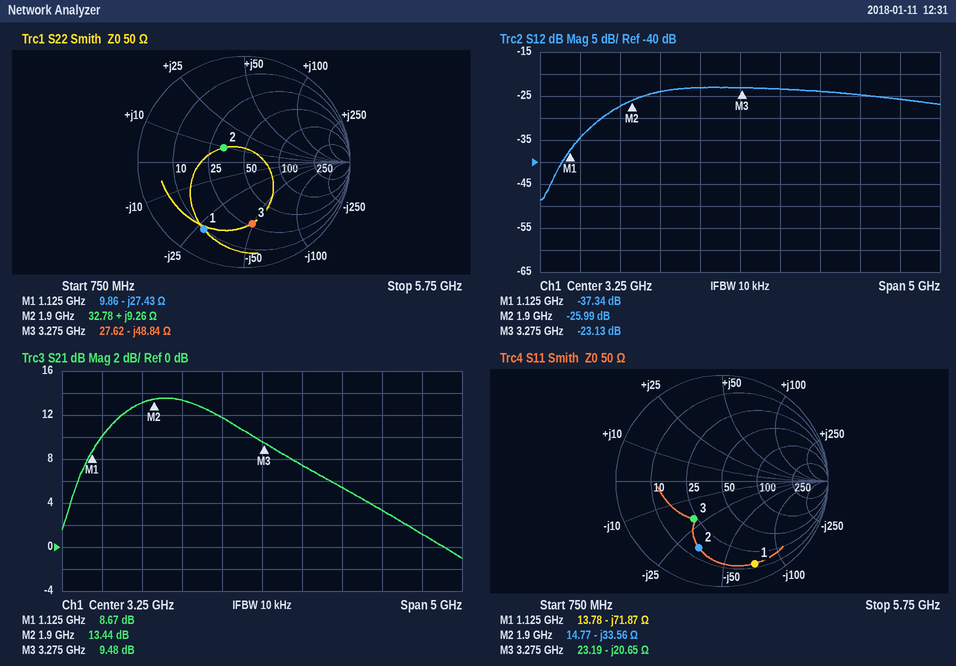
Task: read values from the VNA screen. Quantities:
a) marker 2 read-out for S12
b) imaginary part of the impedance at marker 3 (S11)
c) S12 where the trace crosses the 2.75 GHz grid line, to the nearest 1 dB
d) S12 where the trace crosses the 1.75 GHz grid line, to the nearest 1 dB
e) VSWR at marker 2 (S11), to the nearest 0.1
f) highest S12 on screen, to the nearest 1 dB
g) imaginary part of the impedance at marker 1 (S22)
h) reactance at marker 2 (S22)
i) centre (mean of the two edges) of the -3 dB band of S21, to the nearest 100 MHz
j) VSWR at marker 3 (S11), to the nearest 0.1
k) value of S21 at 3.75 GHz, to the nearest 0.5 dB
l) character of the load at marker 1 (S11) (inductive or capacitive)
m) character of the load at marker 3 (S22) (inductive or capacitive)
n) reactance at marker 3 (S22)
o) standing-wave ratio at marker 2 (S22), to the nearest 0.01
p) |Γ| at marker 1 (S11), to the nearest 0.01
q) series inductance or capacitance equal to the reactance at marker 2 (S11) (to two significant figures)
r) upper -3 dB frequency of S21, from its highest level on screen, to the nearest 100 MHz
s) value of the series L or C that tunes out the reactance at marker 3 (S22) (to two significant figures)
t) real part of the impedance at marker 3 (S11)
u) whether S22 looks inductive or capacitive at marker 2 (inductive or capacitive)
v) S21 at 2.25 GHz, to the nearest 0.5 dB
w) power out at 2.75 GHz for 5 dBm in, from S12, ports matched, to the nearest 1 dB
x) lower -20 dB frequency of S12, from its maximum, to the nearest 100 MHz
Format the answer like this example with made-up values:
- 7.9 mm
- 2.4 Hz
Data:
- -25.99 dB
- -20.65 Ω
- -23 dB
- -27 dB
- 5.0
- -23 dB
- -27.43 Ω
- +9.26 Ω
- 2.2 GHz
- 2.6
- 7.5 dB
- capacitive
- capacitive
- -48.84 Ω
- 1.61
- 0.84
- 2.5 pF
- 3.0 GHz
- 2.4 nH
- 23.19 Ω
- inductive
- 13.5 dB
- -18 dBm
- 900 MHz
